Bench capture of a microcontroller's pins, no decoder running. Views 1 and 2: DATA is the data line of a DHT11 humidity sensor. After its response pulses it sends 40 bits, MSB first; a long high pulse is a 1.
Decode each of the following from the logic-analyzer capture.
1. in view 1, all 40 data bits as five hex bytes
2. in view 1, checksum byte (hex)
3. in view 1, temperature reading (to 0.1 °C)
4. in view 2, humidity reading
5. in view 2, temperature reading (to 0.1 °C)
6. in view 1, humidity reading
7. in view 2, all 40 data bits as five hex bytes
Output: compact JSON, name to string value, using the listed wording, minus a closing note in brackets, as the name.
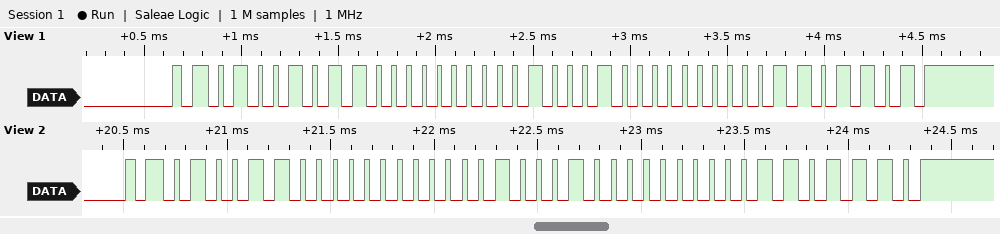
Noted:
{"in view 1, all 40 data bits as five hex bytes": "4B 00 22 00 6D", "in view 1, checksum byte": "0x6D", "in view 1, temperature reading": "34.0 °C", "in view 2, humidity reading": "76 %", "in view 2, temperature reading": "34.0 °C", "in view 1, humidity reading": "75 %", "in view 2, all 40 data bits as five hex bytes": "4C 00 22 00 6E"}
